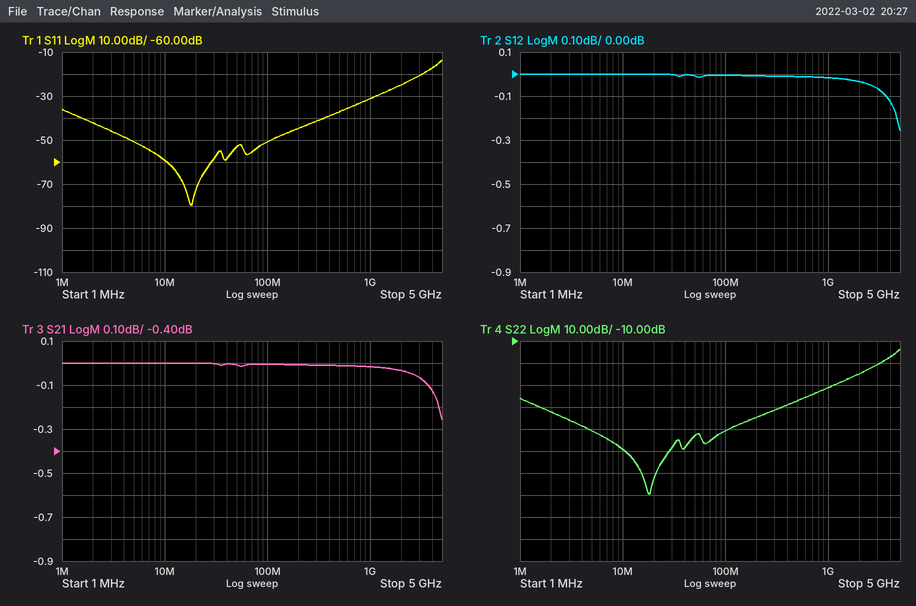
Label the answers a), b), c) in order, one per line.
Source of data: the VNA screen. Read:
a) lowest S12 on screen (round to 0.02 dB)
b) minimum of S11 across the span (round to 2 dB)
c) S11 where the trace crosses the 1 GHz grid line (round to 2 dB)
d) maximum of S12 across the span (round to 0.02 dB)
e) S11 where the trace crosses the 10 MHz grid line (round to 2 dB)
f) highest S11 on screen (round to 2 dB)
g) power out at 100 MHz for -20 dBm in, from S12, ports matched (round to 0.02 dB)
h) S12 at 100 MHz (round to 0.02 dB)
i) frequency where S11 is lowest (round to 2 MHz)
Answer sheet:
a) -0.26 dB
b) -80 dB
c) -32 dB
d) 0.00 dB
e) -60 dB
f) -14 dB
g) -20.00 dBm
h) 0.00 dB
i) 18 MHz
